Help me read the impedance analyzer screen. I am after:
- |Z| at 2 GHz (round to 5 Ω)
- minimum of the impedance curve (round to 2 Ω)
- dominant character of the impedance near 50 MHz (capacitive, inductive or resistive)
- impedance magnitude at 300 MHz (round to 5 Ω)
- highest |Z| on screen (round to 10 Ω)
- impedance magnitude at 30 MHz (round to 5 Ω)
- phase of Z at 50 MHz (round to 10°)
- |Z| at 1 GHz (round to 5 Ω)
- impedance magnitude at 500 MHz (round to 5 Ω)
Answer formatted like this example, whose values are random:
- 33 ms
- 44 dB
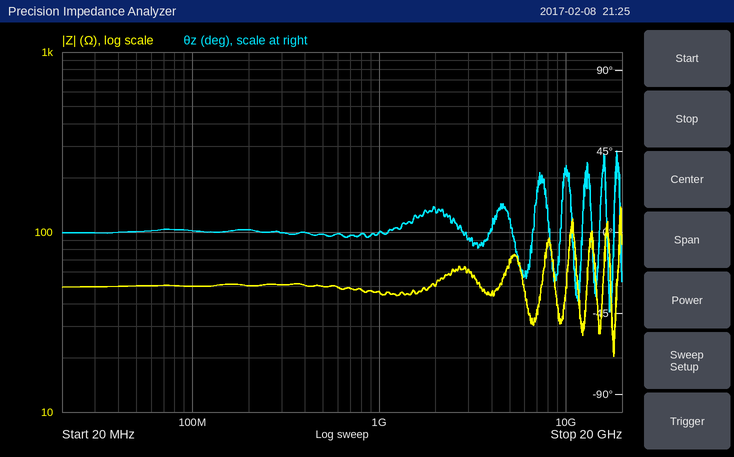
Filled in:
- 50 Ω
- 20 Ω
- resistive
- 50 Ω
- 140 Ω
- 50 Ω
- 0°
- 45 Ω
- 50 Ω
